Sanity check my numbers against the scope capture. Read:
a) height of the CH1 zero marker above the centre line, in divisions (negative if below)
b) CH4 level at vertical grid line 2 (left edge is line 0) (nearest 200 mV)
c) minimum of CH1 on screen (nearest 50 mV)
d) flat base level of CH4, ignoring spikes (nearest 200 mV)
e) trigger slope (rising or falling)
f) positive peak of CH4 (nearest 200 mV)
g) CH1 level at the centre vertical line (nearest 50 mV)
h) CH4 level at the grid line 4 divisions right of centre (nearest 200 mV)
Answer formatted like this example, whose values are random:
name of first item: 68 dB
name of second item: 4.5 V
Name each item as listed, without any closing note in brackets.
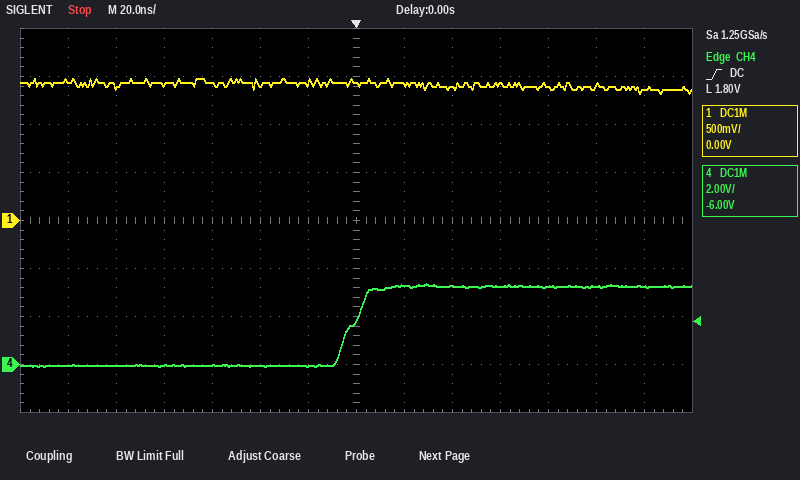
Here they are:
height of the CH1 zero marker above the centre line, in divisions: 0.0 div
CH4 level at vertical grid line 2 (left edge is line 0): 0.0 V
minimum of CH1 on screen: 1.30 V
flat base level of CH4, ignoring spikes: 0.0 V
trigger slope: rising
positive peak of CH4: 3.4 V
CH1 level at the centre vertical line: 1.45 V
CH4 level at the grid line 4 divisions right of centre: 3.2 V
